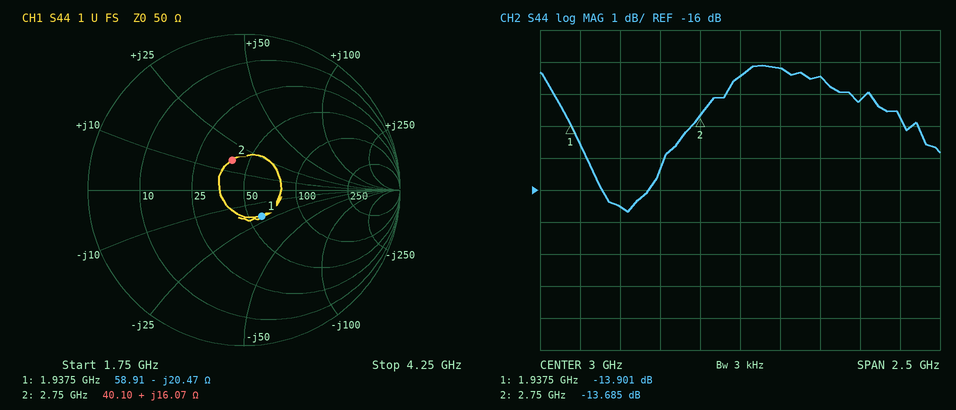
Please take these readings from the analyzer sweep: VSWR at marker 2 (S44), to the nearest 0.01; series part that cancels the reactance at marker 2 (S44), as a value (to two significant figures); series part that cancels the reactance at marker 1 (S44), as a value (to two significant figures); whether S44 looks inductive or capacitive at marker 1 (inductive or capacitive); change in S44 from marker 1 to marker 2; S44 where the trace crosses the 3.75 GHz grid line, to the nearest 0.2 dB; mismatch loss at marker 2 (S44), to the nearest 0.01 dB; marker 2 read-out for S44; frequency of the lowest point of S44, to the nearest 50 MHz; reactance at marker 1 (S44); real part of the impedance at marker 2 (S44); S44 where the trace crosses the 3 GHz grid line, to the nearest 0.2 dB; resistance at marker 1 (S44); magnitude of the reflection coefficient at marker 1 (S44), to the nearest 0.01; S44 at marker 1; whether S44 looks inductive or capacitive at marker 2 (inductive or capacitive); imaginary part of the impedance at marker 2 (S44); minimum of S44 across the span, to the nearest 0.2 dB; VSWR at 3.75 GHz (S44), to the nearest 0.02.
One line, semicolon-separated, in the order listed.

1.52; 3.6 pF; 1.7 nH; capacitive; 0.216 dB; -13.2 dB; 0.19 dB; -13.685 dB; 2.30 GHz; -20.47 Ω; 40.10 Ω; -12.4 dB; 58.91 Ω; 0.20; -13.901 dB; inductive; +16.07 Ω; -16.6 dB; 1.56
